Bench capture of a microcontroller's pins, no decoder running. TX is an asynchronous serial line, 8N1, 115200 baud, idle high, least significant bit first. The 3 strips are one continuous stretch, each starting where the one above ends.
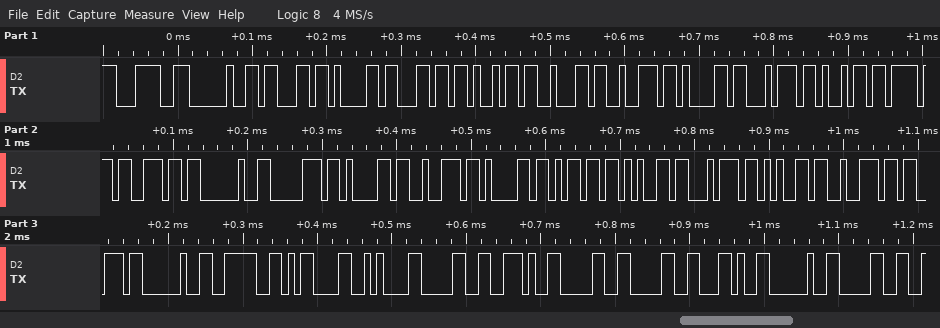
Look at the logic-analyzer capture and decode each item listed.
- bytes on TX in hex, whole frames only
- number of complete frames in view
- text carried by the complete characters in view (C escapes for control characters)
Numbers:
3C 20 63 61 6C 69 62 72 61 74 69 6F 6E 20 70 61 72 61 6D 65 74 65 72 73 20 3E 0D 0A 30 2E 30 30 2C 20 30
35
"< calibration parameters >\r\n0.00, 0"
